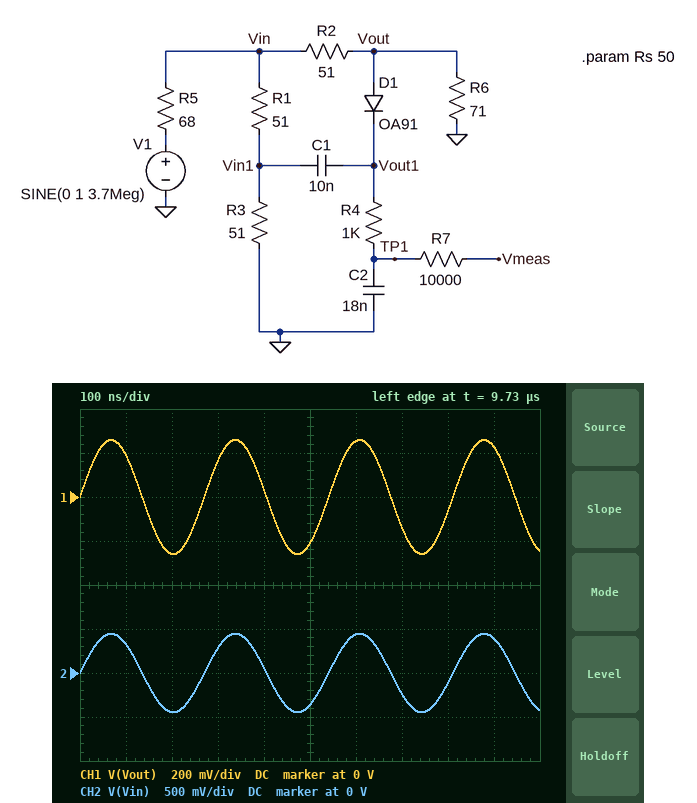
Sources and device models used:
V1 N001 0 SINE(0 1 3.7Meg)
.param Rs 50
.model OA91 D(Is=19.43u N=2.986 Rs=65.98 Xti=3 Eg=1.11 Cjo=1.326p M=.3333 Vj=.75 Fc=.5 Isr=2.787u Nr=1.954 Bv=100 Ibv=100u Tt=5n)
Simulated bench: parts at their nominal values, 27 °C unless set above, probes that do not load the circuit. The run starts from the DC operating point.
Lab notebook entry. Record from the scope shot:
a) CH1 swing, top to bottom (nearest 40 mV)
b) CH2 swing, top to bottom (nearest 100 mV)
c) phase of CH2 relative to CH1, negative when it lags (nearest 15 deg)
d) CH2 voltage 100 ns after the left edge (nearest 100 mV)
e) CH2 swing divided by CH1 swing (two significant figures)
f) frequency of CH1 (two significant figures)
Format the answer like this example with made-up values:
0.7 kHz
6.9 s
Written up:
520 mV
900 mV
0 deg
300 mV
1.7
3.7 MHz
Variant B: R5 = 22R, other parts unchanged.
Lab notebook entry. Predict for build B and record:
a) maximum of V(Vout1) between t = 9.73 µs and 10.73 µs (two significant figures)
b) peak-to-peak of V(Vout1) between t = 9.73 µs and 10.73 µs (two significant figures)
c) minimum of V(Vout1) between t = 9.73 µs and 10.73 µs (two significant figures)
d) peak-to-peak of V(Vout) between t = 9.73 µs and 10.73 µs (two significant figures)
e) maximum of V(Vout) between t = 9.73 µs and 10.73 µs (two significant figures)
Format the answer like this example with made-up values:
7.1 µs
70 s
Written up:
350 mV
700 mV
-350 mV
830 mV
410 mV
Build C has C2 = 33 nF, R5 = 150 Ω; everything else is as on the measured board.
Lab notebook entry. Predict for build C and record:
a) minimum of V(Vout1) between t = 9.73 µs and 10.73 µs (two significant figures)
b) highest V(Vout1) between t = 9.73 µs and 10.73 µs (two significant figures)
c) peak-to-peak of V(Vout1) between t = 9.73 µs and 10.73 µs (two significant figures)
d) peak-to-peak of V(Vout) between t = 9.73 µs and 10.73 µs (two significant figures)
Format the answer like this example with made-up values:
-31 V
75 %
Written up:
-130 mV
130 mV
260 mV
310 mV
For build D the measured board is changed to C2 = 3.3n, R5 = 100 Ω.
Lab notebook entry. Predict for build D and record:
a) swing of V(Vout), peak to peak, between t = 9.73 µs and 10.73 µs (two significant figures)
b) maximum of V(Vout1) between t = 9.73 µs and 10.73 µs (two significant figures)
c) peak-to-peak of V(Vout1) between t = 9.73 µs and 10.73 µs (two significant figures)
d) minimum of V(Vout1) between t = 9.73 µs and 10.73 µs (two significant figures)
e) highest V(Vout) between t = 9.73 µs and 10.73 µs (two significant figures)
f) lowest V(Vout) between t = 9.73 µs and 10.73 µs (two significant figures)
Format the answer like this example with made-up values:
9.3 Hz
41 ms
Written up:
410 mV
170 mV
350 mV
-170 mV
210 mV
-210 mV
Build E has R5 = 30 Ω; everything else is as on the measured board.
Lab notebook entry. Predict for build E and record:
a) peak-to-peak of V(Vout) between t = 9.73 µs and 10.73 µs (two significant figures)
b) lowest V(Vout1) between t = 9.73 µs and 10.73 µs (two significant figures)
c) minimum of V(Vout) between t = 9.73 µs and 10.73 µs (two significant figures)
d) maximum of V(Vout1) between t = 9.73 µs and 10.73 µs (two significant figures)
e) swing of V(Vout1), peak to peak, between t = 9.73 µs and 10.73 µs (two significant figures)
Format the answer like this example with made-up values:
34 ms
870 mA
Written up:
750 mV
-310 mV
-380 mV
320 mV
630 mV
